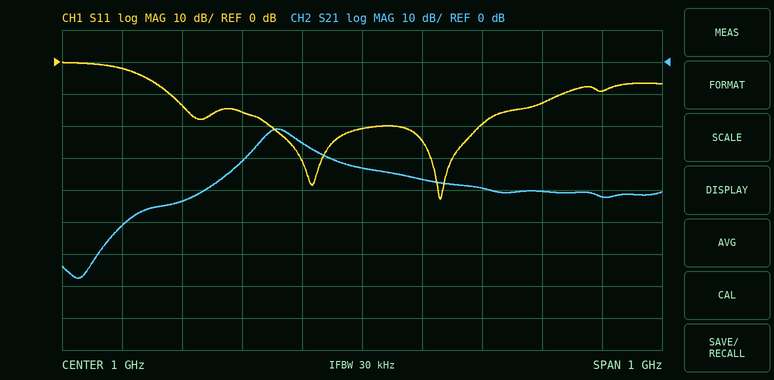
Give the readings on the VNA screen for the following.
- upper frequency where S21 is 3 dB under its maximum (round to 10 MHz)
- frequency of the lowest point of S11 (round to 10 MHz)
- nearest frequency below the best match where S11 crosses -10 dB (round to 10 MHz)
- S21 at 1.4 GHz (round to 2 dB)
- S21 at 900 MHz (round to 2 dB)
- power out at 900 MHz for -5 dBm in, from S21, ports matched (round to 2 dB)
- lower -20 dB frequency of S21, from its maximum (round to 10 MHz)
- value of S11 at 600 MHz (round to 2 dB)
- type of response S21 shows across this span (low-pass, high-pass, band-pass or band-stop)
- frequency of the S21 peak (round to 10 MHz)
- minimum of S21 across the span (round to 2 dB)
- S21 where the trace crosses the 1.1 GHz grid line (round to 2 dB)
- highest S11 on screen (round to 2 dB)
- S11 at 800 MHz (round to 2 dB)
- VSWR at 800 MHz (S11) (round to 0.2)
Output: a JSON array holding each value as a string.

["890 MHz", "1.13 GHz", "680 MHz", "-42 dB", "-26 dB", "-30 dBm", "730 MHz", "-2 dB", "band-pass", "860 MHz", "-68 dB", "-36 dB", "0 dB", "-16 dB", "1.4"]
